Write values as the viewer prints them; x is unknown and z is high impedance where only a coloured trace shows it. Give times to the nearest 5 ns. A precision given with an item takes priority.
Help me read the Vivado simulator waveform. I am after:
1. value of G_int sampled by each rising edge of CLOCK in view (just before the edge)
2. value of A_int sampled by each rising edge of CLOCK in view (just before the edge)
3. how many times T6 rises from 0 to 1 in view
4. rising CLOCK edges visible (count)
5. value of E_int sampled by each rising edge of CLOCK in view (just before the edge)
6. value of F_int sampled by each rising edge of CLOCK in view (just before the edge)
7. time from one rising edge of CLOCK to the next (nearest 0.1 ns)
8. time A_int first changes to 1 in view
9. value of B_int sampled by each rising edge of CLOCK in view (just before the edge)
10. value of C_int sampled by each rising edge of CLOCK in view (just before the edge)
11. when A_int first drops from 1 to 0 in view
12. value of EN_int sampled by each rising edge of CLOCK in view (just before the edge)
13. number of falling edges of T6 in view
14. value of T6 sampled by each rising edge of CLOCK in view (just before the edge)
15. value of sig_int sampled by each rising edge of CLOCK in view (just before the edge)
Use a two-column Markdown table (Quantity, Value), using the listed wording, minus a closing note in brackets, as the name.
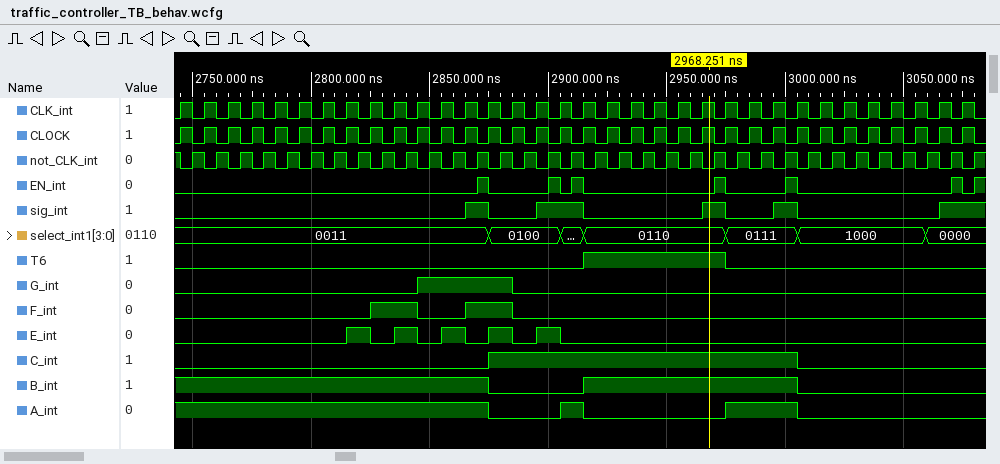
| Quantity | Value |
|---|---|
| value of G_int sampled by each rising edge of CLOCK in view | 0 0 0 0 0 0 0 0 0 0 0 1 1 1 1 0 0 0 0 0 0 0 0 0 0 0 0 0 0 0 0 0 0 0 |
| value of A_int sampled by each rising edge of CLOCK in view | 1 1 1 1 1 1 1 1 1 1 1 1 1 1 0 0 0 1 0 0 0 0 0 0 1 1 1 0 0 0 0 0 0 0 |
| how many times T6 rises from 0 to 1 in view | 1 |
| rising CLOCK edges visible | 34 |
| value of E_int sampled by each rising edge of CLOCK in view | 0 0 0 0 0 0 0 0 1 0 1 0 1 0 1 0 1 0 0 0 0 0 0 0 0 0 0 0 0 0 0 0 0 0 |
| value of F_int sampled by each rising edge of CLOCK in view | 0 0 0 0 0 0 0 0 0 1 1 0 0 1 1 0 0 0 0 0 0 0 0 0 0 0 0 0 0 0 0 0 0 0 |
| time from one rising edge of CLOCK to the next | 10 ns |
| time A_int first changes to 1 in view | 2905 ns |
| value of B_int sampled by each rising edge of CLOCK in view | 1 1 1 1 1 1 1 1 1 1 1 1 1 1 0 0 0 0 1 1 1 1 1 1 1 1 1 0 0 0 0 0 0 0 |
| value of C_int sampled by each rising edge of CLOCK in view | 0 0 0 0 0 0 0 0 0 0 0 0 0 0 1 1 1 1 1 1 1 1 1 1 1 1 1 0 0 0 0 0 0 0 |
| when A_int first drops from 1 to 0 in view | 2875 ns |
| value of EN_int sampled by each rising edge of CLOCK in view | 0 0 0 0 0 0 0 0 0 0 0 0 0 1 0 0 1 1 0 0 0 0 0 1 0 0 1 0 0 0 0 0 0 1 |
| number of falling edges of T6 in view | 1 |
| value of T6 sampled by each rising edge of CLOCK in view | 0 0 0 0 0 0 0 0 0 0 0 0 0 0 0 0 0 0 1 1 1 1 1 1 0 0 0 0 0 0 0 0 0 0 |
| value of sig_int sampled by each rising edge of CLOCK in view | 0 0 0 0 0 0 0 0 0 0 0 0 0 1 0 0 1 1 0 0 0 0 0 1 0 0 1 0 0 0 0 0 0 1 |
